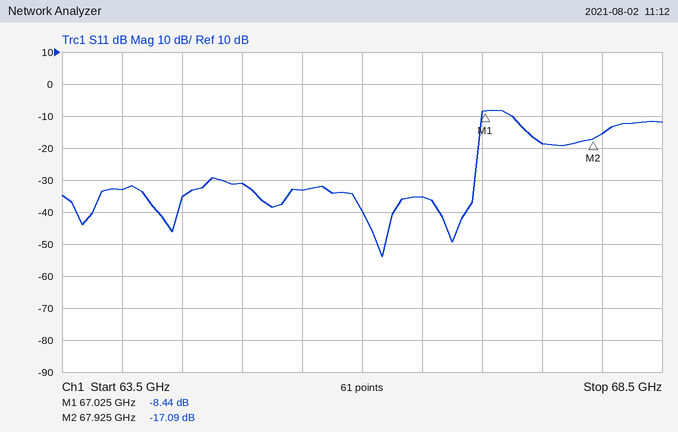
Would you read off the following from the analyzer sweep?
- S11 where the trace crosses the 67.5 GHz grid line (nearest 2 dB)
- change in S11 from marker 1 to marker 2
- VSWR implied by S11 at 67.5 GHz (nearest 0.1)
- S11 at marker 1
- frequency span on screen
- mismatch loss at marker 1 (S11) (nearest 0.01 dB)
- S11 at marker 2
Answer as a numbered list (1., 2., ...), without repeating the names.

1. -18 dB
2. -8.65 dB
3. 1.3
4. -8.44 dB
5. 5 GHz
6. 0.67 dB
7. -17.09 dB
